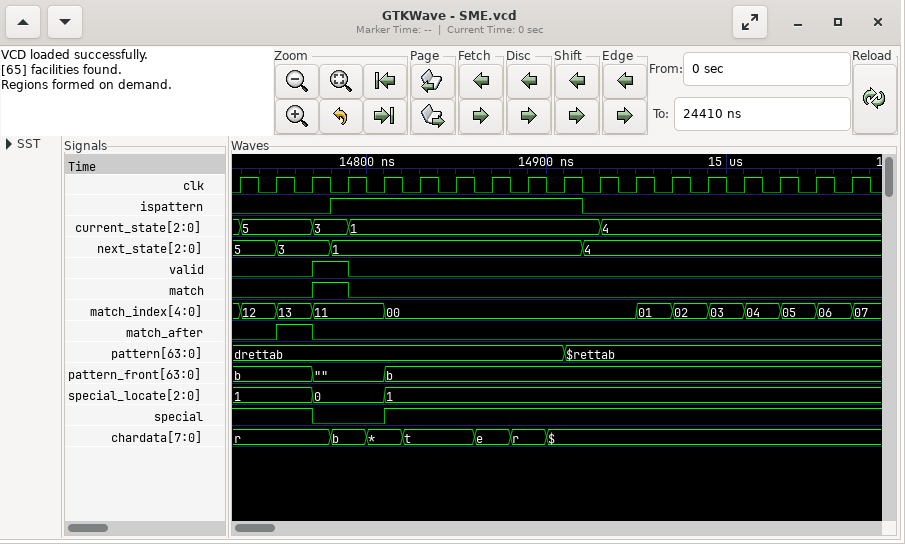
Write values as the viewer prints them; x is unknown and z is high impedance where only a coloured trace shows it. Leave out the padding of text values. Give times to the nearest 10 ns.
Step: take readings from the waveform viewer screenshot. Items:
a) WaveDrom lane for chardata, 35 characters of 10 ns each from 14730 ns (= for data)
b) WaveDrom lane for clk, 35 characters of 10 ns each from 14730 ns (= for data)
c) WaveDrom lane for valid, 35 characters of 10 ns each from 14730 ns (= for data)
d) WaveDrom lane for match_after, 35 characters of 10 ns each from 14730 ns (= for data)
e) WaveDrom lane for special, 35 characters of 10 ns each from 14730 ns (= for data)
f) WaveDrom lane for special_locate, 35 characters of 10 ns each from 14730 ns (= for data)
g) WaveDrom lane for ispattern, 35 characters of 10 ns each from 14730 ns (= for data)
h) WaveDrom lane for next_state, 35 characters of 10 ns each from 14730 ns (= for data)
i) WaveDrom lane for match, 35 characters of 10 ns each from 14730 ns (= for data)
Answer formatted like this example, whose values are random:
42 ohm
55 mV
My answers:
{name: 'chardata', wave: '=....=.=.=...=.=.=.................', data: 'r b * t e r $'}
{name: 'clk', wave: '10101010101010101010101010101010101'}
{name: 'valid', wave: '0...1.0............................'}
{name: 'match_after', wave: '0.1.0..............................'}
{name: 'special', wave: '1...0...1..........................'}
{name: 'special_locate', wave: '=...=...=..........................', data: '1 0 1'}
{name: 'ispattern', wave: '0....1.............0...............'}
{name: 'next_state', wave: '=.=..=.............=...............', data: '5 3 1 4'}
{name: 'match', wave: '0...1.0............................'}
